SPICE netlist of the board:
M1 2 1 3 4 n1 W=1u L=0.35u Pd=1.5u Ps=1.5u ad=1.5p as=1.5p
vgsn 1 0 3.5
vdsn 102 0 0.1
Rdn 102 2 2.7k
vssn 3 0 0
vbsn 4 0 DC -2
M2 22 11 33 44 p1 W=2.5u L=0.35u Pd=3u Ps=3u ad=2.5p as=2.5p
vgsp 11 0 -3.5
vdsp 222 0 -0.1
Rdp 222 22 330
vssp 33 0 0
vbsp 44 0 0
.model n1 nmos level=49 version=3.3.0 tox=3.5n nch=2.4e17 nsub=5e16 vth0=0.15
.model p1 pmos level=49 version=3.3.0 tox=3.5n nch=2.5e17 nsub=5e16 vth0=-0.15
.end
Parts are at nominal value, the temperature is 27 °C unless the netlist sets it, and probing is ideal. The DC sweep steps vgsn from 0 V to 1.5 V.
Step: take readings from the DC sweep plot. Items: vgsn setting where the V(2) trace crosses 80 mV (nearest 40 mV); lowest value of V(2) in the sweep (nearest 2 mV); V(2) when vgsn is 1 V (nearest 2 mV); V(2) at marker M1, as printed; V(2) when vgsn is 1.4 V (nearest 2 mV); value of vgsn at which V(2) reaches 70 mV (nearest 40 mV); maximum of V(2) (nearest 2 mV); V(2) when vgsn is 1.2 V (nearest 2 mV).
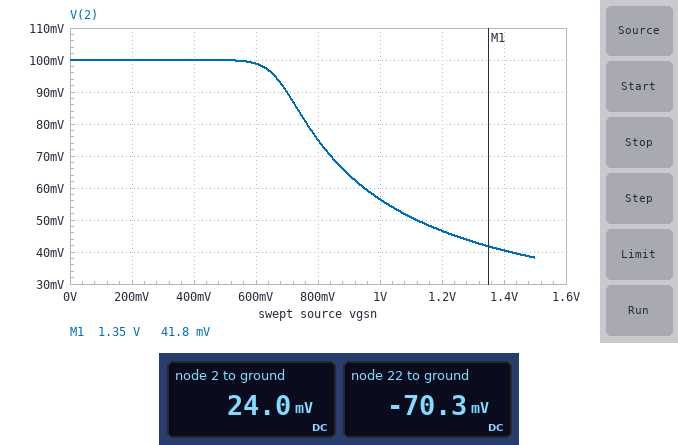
760 mV
38 mV
56 mV
41.8 mV
40 mV
840 mV
100 mV
46 mV
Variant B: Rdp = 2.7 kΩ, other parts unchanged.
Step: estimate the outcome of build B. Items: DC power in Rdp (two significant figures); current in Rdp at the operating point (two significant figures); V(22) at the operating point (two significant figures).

2.2 µW
29 µA
-22 mV
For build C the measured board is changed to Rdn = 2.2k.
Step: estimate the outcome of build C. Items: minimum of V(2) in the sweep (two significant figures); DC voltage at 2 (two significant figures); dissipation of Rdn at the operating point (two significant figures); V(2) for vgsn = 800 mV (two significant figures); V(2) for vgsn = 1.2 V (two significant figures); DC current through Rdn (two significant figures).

43 mV
28 mV
2.4 µW
79 mV
52 mV
33 µA
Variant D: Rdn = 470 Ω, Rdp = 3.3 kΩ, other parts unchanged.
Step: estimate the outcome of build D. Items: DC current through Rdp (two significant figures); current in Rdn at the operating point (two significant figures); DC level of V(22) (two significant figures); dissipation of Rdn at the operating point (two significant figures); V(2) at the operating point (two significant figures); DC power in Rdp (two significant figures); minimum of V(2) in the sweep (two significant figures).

25 µA
75 µA
-19 mV
2.6 µW
65 mV
2.0 µW
79 mV
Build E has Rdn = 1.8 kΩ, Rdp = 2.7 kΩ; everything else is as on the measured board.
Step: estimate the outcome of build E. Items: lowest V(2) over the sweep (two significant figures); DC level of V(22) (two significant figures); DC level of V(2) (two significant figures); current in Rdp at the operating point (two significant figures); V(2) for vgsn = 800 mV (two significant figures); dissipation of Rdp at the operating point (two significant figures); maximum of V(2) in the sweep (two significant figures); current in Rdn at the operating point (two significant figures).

48 mV
-22 mV
32 mV
29 µA
82 mV
2.2 µW
100 mV
38 µA
